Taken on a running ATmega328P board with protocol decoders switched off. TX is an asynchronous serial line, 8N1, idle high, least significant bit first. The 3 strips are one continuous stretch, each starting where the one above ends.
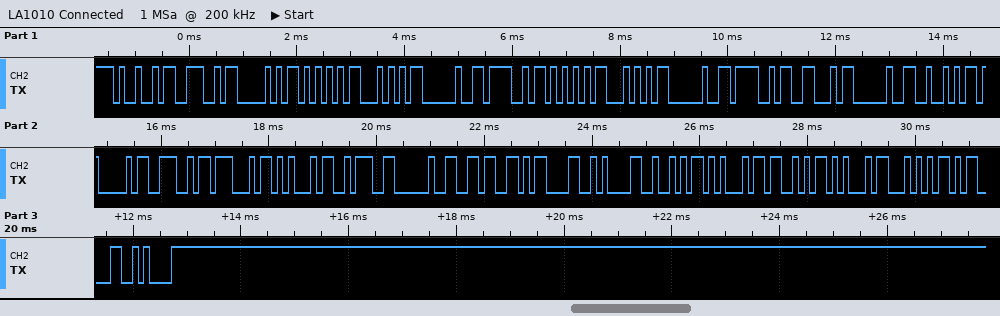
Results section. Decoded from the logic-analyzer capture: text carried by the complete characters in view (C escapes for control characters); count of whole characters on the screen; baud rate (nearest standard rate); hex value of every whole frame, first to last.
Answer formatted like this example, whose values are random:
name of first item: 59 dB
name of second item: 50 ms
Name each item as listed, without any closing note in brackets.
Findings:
text carried by the complete characters in view: "INPUT OUT OF RANGE: 6\r\nRESET\r\n"
count of whole characters on the screen: 30
baud rate: 9600 baud
hex value of every whole frame, first to last: 49 4E 50 55 54 20 4F 55 54 20 4F 46 20 52 41 4E 47 45 3A 20 36 0D 0A 52 45 53 45 54 0D 0A
